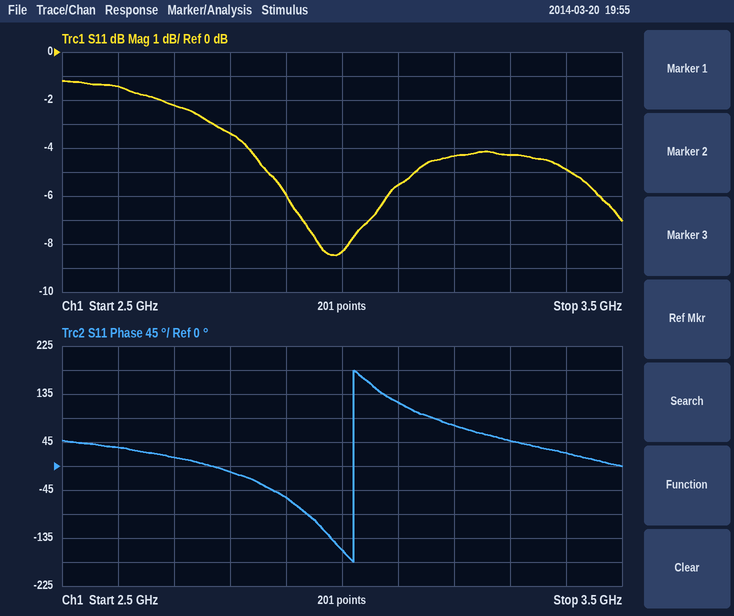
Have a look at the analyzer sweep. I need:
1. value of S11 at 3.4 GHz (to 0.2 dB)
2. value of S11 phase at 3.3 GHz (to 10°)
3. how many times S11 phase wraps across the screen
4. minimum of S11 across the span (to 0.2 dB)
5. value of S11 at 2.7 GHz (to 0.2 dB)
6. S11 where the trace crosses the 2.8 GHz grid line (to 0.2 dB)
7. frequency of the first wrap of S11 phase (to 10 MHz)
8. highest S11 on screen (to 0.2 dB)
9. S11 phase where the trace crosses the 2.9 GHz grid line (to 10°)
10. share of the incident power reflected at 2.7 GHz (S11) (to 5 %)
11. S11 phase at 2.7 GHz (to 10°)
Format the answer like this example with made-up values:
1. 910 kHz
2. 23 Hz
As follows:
1. -4.8 dB
2. 50°
3. 1
4. -8.4 dB
5. -2.2 dB
6. -3.4 dB
7. 3.02 GHz
8. -1.2 dB
9. -60°
10. 60 %
11. 20°
